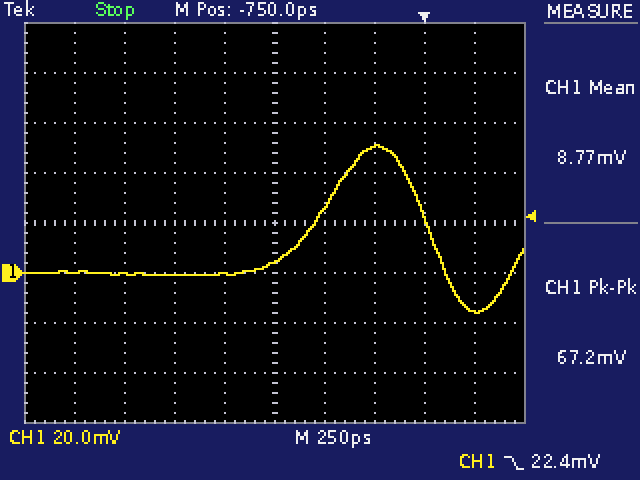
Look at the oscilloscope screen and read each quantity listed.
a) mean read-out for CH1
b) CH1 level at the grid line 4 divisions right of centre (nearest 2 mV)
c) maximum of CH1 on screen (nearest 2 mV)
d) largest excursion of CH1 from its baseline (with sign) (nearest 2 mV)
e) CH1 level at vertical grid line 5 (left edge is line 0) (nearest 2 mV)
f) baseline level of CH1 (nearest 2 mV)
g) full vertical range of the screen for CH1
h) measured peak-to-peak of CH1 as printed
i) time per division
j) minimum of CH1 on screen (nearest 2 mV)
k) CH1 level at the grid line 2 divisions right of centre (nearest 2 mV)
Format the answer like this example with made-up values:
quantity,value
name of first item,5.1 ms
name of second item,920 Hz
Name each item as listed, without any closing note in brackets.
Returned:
quantity,value
mean read-out for CH1,8.77 mV
CH1 level at the grid line 4 divisions right of centre,-16 mV
maximum of CH1 on screen,52 mV
largest excursion of CH1 from its baseline (with sign),+52 mV
CH1 level at vertical grid line 5 (left edge is line 0),4 mV
baseline level of CH1,0 mV
full vertical range of the screen for CH1,160 mV
measured peak-to-peak of CH1 as printed,67.2 mV
time per division,250 ps
minimum of CH1 on screen,-16 mV
CH1 level at the grid line 2 divisions right of centre,50 mV
